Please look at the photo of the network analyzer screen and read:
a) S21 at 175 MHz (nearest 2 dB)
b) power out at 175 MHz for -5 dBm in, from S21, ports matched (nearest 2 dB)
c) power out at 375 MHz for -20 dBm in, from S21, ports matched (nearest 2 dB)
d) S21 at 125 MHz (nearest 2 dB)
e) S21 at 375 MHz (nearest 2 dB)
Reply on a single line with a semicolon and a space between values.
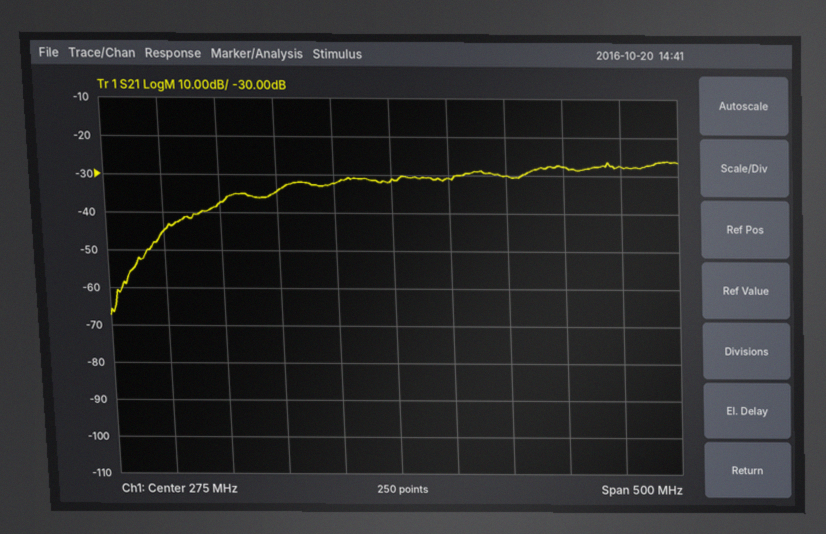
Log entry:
-34 dB; -40 dBm; -50 dBm; -38 dB; -30 dB
